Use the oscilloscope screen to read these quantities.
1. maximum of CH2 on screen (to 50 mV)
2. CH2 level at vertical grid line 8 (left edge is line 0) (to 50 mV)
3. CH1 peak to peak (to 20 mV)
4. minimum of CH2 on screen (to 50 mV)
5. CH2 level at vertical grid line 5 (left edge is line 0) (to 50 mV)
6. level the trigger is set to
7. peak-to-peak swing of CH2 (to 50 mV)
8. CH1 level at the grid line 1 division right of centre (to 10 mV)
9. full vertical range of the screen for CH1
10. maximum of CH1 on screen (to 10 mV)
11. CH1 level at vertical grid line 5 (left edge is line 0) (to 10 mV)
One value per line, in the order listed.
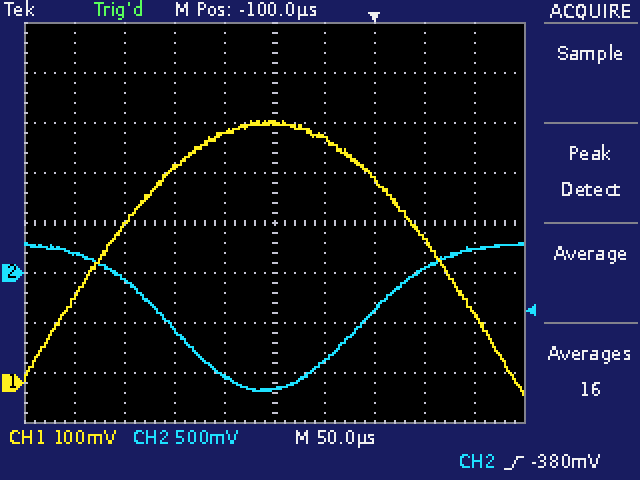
300 mV
50 mV
540 mV
-1.20 V
-1.15 V
-380 mV
1.50 V
490 mV
800 mV
520 mV
520 mV
